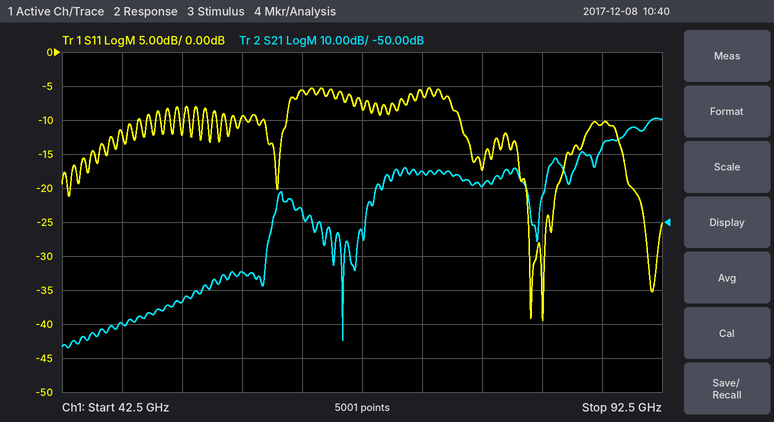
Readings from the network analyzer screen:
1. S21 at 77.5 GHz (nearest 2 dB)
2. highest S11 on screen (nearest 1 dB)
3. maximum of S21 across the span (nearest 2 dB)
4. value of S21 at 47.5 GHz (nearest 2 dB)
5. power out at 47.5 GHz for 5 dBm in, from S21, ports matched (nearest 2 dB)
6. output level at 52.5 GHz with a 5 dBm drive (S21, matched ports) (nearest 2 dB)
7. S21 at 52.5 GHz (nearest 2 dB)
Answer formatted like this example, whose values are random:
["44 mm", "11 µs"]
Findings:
["-40 dB", "-5 dB", "-20 dB", "-80 dB", "-74 dBm", "-68 dBm", "-74 dB"]
